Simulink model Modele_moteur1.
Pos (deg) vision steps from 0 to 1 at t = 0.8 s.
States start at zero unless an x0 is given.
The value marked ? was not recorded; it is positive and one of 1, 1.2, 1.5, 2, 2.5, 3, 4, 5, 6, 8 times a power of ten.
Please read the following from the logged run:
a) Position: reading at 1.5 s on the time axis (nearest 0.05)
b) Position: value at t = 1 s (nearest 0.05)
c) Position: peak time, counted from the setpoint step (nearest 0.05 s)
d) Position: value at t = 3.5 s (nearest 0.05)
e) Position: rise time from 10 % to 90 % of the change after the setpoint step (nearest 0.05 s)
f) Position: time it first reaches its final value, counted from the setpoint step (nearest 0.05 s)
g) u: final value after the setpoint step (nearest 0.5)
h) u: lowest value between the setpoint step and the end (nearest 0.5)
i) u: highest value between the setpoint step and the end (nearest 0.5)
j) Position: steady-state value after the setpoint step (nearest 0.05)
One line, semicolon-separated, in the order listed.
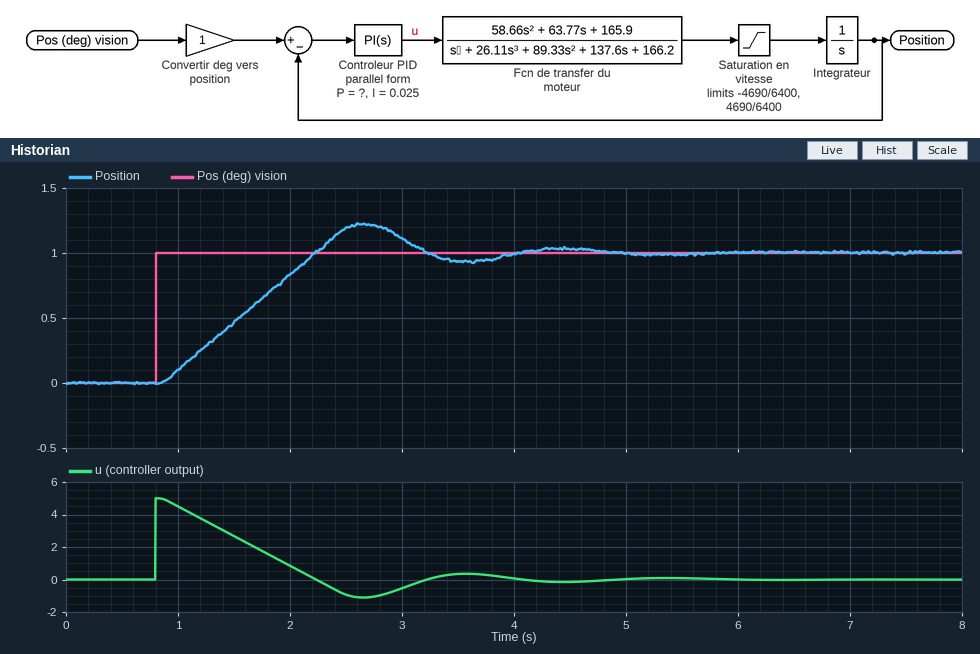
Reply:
0.45; 0.10; 1.85 s; 0.95; 1.10 s; 1.45 s; 0.0; -1.0; 5.0; 1.00
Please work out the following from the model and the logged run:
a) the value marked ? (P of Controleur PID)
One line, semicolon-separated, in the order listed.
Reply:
5
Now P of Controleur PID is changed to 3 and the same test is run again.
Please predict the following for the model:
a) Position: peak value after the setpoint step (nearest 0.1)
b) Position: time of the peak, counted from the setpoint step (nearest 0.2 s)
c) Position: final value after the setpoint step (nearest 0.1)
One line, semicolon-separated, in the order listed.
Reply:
1.2; 2.0 s; 1.0
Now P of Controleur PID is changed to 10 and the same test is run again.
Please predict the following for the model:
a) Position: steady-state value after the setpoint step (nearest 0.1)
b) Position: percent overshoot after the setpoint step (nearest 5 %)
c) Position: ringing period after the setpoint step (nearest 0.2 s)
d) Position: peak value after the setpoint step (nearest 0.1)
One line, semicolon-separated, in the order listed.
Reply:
1.0; 25 %; 1.4 s; 1.3
